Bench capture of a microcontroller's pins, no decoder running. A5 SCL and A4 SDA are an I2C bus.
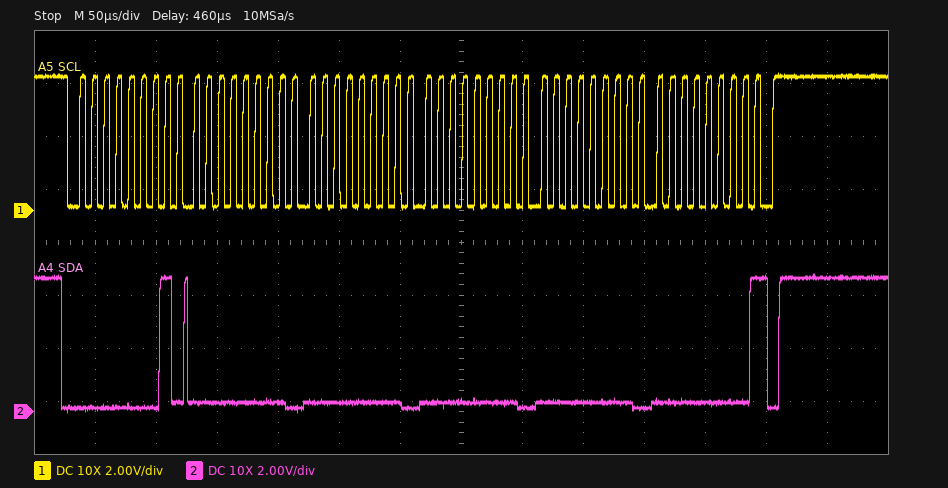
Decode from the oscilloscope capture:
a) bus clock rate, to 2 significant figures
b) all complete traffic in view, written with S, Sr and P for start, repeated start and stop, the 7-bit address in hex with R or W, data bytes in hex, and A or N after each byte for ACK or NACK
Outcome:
100 kHz
S 00R A 00 A 00 A 00 A 00 A 00 N P
